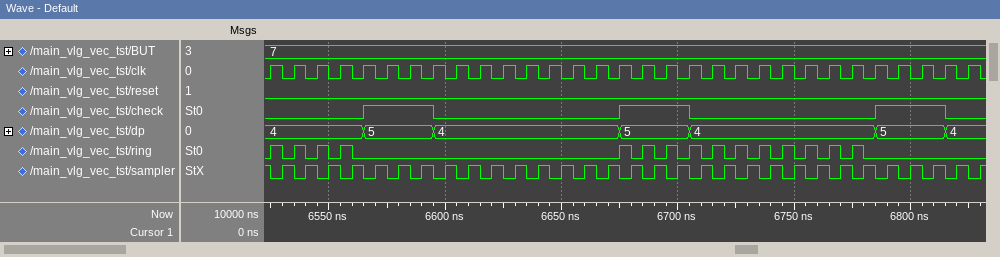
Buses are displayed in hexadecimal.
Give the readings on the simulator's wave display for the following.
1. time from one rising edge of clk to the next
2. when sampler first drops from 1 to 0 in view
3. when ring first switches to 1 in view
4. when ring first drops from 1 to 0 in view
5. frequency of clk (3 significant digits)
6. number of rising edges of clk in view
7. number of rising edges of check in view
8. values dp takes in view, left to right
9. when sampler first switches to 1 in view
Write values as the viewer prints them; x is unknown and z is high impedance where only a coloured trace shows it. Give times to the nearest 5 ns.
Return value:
10 ns
6525 ns
6525 ns
6530 ns
100 MHz
31
3
4, 5, 4, 5, 4, 5, 4
6530 ns
